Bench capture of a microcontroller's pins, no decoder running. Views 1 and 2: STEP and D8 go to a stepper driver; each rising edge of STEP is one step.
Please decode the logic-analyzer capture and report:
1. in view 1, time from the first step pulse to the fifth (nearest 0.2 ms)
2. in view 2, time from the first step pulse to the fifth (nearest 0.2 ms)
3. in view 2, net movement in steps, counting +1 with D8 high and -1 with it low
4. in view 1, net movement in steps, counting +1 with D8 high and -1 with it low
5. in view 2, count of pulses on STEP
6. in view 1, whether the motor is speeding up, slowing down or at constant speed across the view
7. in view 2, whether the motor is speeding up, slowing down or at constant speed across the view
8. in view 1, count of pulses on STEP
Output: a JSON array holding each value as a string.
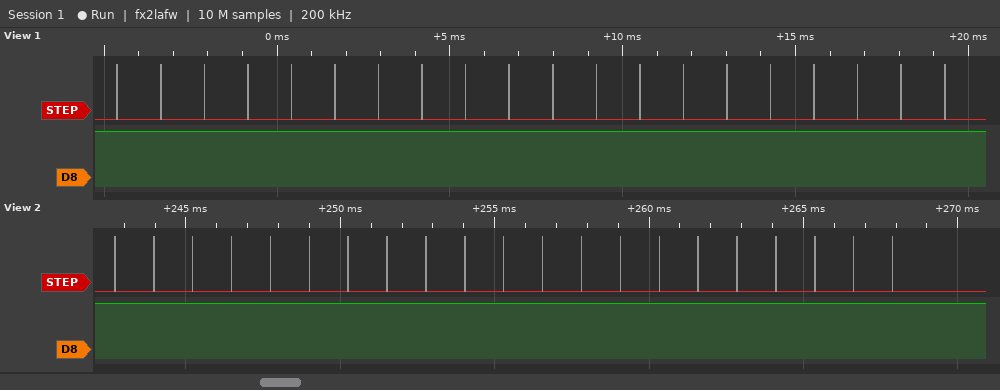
["5.0 ms", "5.0 ms", "+21", "+20", "21", "constant speed", "constant speed", "20"]
